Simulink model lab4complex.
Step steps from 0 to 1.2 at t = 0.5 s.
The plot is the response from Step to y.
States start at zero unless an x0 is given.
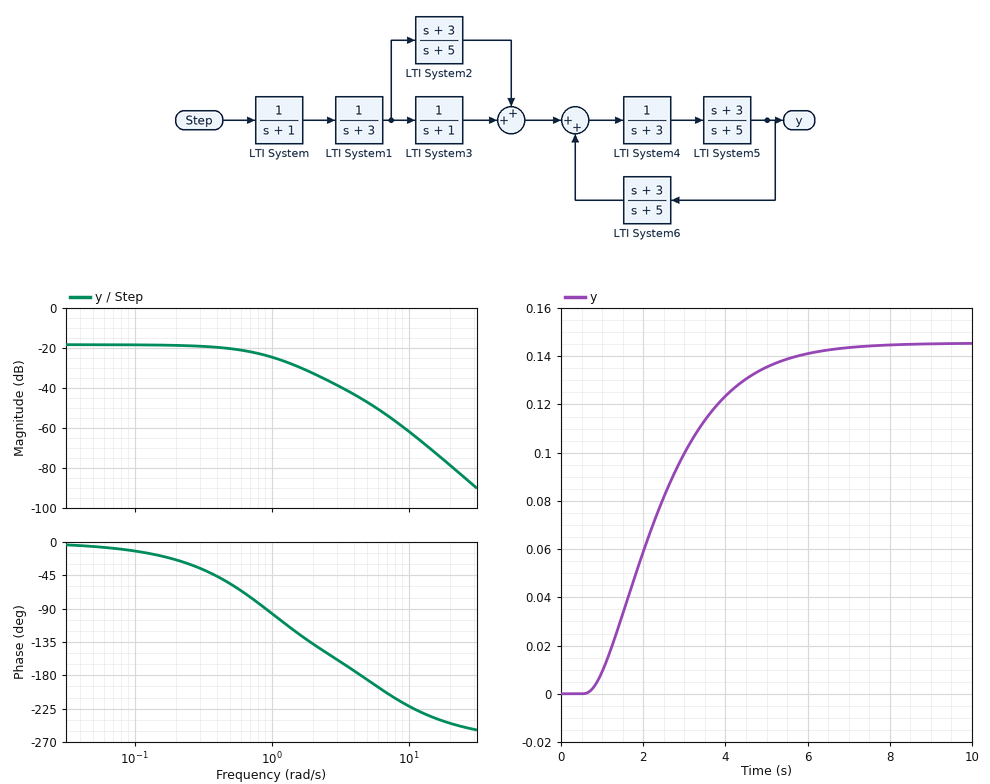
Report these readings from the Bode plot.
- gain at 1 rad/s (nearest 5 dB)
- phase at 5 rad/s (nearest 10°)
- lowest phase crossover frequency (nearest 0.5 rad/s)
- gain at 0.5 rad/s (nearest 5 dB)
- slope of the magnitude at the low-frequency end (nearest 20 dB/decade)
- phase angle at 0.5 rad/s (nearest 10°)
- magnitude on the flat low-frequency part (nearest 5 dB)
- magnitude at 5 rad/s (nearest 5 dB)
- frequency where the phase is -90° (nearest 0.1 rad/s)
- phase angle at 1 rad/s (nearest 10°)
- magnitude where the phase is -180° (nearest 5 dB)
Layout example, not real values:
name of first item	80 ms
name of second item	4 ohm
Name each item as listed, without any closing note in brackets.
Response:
gain at 1 rad/s	-25 dB
phase at 5 rad/s	-190°
lowest phase crossover frequency	4.5 rad/s
gain at 0.5 rad/s	-20 dB
slope of the magnitude at the low-frequency end	0 dB/decade
phase angle at 0.5 rad/s	-60°
magnitude on the flat low-frequency part	-20 dB
magnitude at 5 rad/s	-45 dB
frequency where the phase is -90°	0.9 rad/s
phase angle at 1 rad/s	-100°
magnitude where the phase is -180°	-45 dB
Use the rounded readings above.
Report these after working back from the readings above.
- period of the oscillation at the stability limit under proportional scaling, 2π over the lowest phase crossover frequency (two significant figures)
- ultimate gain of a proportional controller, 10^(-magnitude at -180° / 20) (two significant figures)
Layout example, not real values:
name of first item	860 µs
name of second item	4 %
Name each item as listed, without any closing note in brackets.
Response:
period of the oscillation at the stability limit under proportional scaling, 2π over the lowest phase crossover frequency	1.4 s
ultimate gain of a proportional controller, 10^(-magnitude at -180° / 20)	180
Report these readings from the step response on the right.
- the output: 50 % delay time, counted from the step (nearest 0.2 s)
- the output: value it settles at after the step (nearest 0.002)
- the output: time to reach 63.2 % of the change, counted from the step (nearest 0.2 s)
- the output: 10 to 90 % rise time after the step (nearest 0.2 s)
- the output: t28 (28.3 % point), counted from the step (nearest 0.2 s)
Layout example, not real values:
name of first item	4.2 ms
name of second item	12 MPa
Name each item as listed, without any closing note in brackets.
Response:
the output: 50 % delay time, counted from the step	1.8 s
the output: value it settles at after the step	0.146
the output: time to reach 63.2 % of the change, counted from the step	2.2 s
the output: 10 to 90 % rise time after the step	3.4 s
the output: t28 (28.3 % point), counted from the step	1.2 s
